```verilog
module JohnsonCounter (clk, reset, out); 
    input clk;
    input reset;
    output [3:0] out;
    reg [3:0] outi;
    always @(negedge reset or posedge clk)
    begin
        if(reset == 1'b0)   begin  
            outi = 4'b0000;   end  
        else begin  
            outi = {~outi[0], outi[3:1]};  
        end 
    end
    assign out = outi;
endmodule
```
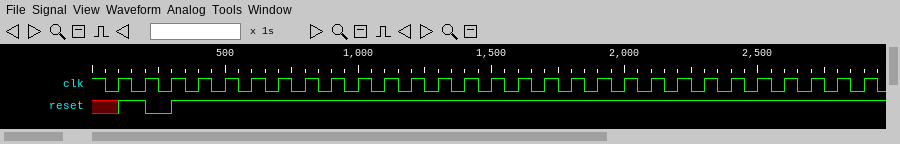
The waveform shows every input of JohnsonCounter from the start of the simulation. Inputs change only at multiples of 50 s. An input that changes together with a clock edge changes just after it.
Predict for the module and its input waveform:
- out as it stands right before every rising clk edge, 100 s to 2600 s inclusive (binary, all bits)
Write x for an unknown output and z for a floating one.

x, x, 0000, 0000, 1000, 1100, 1110, 1111, 0111, 0011, 0001, 0000, 1000, 1100, 1110, 1111, 0111, 0011, 0001, 0000, 1000, 1100, 1110, 1111, 0111, 0011
